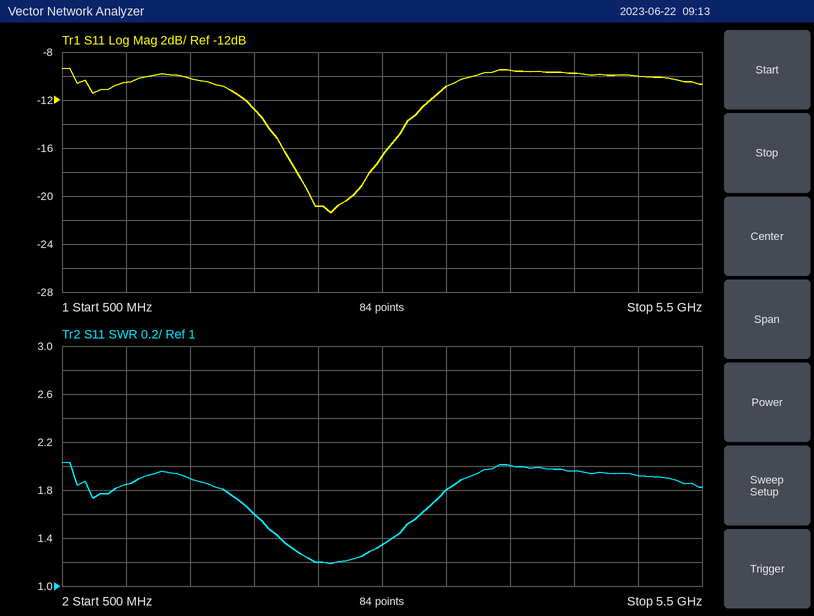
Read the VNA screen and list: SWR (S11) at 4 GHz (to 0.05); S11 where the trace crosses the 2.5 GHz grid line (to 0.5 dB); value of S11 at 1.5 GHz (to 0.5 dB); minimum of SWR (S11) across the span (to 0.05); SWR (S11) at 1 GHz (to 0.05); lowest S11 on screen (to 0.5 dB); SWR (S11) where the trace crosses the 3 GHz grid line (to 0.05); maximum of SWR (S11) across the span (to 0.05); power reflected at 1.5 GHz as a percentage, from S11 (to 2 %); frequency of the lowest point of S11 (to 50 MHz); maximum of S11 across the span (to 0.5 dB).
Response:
2.00
-21.0 dB
-10.0 dB
1.20
1.85
-21.5 dB
1.35
2.05
10 %
2.60 GHz
-9.5 dB
